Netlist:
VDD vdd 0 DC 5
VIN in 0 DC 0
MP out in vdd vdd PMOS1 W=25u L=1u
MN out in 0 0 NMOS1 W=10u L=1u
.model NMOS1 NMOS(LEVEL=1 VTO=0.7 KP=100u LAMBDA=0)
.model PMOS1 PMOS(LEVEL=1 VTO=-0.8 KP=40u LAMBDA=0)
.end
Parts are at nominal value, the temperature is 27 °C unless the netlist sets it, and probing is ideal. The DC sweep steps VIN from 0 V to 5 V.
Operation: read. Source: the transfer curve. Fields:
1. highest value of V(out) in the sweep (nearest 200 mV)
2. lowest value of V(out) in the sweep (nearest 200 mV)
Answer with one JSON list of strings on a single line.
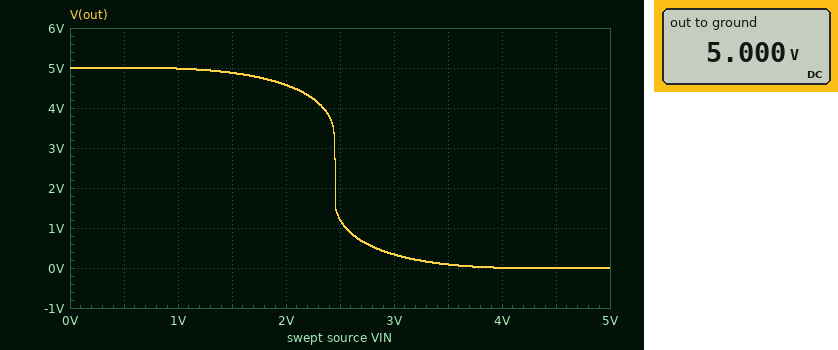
["5.0 V", "0 V"]
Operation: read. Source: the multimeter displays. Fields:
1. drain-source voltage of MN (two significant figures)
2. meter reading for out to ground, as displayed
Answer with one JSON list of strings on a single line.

["5.0 V", "5.000 V"]
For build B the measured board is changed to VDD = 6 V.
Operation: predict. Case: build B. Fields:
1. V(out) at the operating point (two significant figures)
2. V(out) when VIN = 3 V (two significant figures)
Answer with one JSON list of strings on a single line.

["6.0 V", "1.6 V"]
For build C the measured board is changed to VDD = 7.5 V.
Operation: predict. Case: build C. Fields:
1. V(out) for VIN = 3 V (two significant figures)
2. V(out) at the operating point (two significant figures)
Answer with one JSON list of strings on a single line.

["6.7 V", "7.5 V"]
